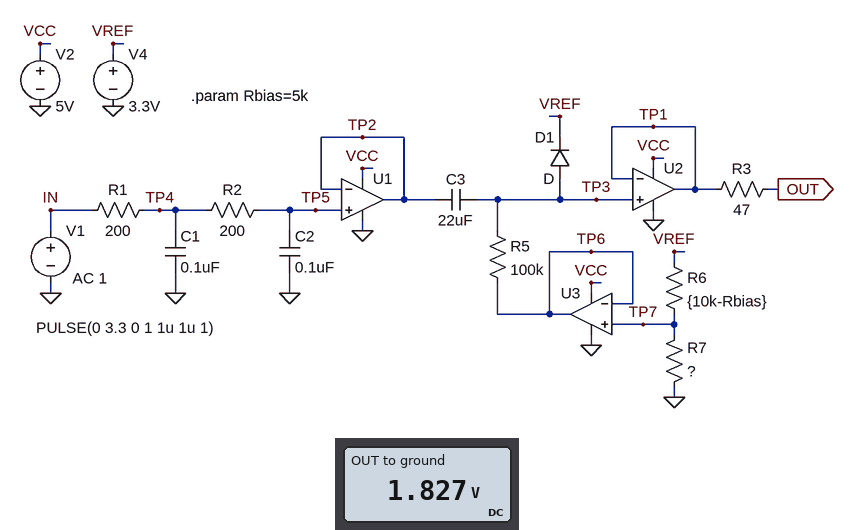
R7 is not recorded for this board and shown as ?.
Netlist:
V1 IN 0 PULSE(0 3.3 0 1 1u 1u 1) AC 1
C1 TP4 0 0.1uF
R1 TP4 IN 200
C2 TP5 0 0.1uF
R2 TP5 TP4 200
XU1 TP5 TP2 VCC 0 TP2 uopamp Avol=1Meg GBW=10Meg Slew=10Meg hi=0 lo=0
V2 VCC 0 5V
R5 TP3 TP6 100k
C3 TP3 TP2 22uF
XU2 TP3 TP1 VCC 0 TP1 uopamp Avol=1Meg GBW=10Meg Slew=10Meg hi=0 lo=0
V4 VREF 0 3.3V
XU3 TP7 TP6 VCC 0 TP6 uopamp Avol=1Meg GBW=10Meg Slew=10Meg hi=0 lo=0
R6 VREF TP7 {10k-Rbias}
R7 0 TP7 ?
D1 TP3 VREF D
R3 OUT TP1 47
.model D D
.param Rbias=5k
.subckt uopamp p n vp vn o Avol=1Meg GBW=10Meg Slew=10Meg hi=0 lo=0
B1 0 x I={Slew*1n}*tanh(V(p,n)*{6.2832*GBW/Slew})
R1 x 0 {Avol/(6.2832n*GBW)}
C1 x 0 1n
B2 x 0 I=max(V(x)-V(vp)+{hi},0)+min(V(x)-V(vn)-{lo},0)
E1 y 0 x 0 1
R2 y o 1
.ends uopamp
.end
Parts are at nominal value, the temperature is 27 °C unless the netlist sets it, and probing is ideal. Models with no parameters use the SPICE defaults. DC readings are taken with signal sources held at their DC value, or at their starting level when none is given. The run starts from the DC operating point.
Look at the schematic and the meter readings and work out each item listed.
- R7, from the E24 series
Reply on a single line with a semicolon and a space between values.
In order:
6.2 kΩ
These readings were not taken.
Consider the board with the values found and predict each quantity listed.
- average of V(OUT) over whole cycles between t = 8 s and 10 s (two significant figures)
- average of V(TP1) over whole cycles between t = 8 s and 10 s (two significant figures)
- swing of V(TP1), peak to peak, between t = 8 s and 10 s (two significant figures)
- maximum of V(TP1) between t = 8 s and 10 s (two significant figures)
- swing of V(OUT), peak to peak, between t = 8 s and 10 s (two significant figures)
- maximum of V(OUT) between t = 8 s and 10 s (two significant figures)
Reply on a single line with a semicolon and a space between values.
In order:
1.8 V; 1.8 V; 3.3 V; 3.4 V; 3.3 V; 3.4 V
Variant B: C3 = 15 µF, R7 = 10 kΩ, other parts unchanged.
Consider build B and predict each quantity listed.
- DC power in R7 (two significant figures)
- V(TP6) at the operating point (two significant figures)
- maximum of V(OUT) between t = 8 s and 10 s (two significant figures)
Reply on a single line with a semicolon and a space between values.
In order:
480 µW; 2.2 V; 3.7 V
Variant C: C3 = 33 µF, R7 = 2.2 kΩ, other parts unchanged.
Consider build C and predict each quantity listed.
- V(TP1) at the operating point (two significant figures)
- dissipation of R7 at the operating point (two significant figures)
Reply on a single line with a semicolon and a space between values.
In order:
1.0 V; 460 µW
